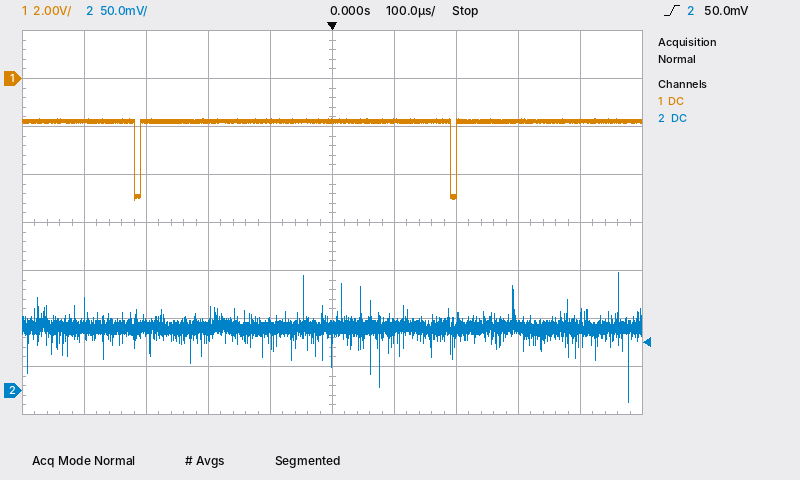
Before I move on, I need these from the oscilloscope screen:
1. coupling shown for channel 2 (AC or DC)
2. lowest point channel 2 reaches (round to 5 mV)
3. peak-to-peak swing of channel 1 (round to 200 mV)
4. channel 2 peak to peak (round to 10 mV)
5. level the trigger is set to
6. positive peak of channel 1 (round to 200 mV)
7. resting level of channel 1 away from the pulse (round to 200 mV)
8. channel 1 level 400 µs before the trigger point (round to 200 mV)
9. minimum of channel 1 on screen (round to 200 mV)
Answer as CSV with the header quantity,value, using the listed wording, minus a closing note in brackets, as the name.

quantity,value
coupling shown for channel 2,DC
lowest point channel 2 reaches,-10 mV
peak-to-peak swing of channel 1,3.4 V
channel 2 peak to peak,130 mV
level the trigger is set to,50.0 mV
positive peak of channel 1,-1.6 V
resting level of channel 1 away from the pulse,-1.8 V
channel 1 level 400 µs before the trigger point,-1.8 V
minimum of channel 1 on screen,-5.0 V
